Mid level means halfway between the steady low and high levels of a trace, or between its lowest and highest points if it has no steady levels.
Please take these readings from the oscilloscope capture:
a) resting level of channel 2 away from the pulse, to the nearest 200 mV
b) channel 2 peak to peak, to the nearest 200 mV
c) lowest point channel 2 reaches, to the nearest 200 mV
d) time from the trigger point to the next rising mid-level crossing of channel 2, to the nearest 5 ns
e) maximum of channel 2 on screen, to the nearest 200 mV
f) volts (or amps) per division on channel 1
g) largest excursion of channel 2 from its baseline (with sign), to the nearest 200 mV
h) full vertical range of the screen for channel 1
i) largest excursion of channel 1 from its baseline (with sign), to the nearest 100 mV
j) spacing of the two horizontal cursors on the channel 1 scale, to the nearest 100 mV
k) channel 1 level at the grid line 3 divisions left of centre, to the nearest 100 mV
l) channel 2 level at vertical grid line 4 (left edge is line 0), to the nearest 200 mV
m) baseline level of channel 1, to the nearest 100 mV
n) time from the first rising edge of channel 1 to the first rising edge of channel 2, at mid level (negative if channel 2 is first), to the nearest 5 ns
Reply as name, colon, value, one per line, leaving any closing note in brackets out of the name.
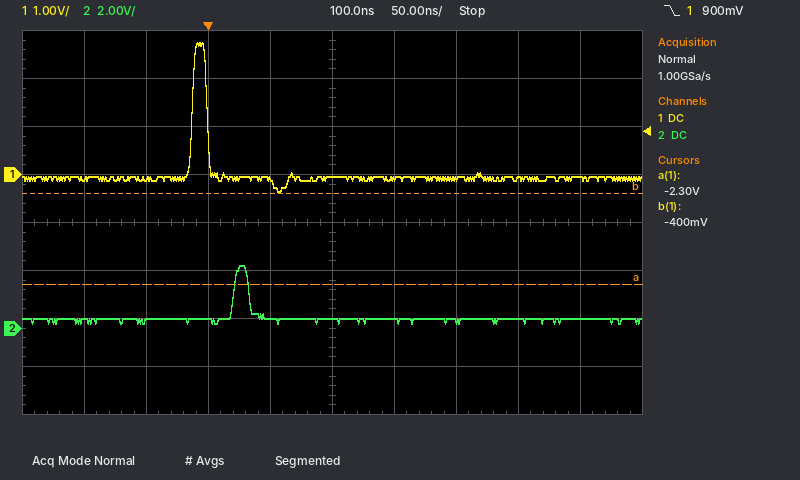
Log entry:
resting level of channel 2 away from the pulse, to the nearest 200 mV: 400 mV
channel 2 peak to peak, to the nearest 200 mV: 2.4 V
lowest point channel 2 reaches, to the nearest 200 mV: 200 mV
time from the trigger point to the next rising mid-level crossing of channel 2, to the nearest 5 ns: 20 ns
maximum of channel 2 on screen, to the nearest 200 mV: 2.6 V
volts (or amps) per division on channel 1: 1 V
largest excursion of channel 2 from its baseline (with sign), to the nearest 200 mV: +2.2 V
full vertical range of the screen for channel 1: 8 V
largest excursion of channel 1 from its baseline (with sign), to the nearest 100 mV: +2.8 V
spacing of the two horizontal cursors on the channel 1 scale, to the nearest 100 mV: 1.9 V
channel 1 level at the grid line 3 divisions left of centre, to the nearest 100 mV: -100 mV
channel 2 level at vertical grid line 4 (left edge is line 0), to the nearest 200 mV: 400 mV
baseline level of channel 1, to the nearest 100 mV: -100 mV
time from the first rising edge of channel 1 to the first rising edge of channel 2, at mid level (negative if channel 2 is first), to the nearest 5 ns: +35 ns
